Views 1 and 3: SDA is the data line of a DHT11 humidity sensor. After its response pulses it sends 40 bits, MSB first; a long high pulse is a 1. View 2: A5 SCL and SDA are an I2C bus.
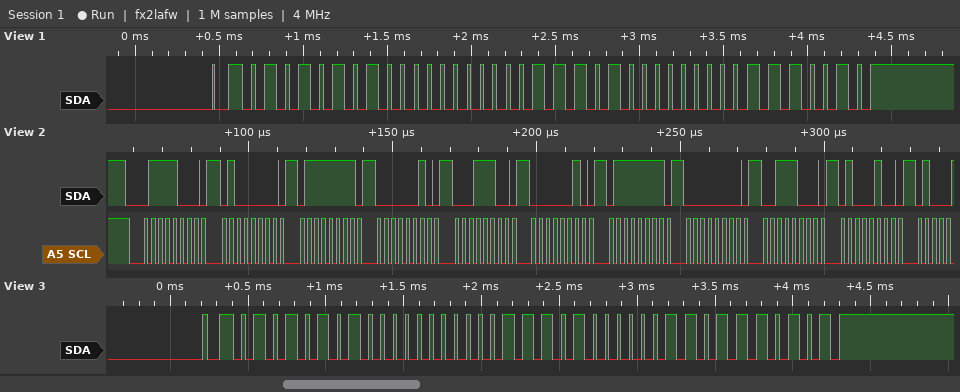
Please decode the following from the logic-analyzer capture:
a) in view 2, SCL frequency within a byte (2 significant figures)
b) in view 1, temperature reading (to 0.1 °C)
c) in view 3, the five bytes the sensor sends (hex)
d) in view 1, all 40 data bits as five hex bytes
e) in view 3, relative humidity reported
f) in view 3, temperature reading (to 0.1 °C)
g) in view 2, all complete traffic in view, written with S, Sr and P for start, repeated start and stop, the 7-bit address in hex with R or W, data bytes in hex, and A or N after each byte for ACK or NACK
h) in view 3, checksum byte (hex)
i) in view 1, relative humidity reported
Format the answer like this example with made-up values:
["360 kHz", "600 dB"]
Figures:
["400 kHz", "29.0 °C", "55 00 1D 03 75", "55 00 1D 00 72", "85 %", "29.3 °C", "S 3CW A 40 A 7F A 02 A 1C A 02 A 7F A 00 A 38 A 44 A", "0x75", "85 %"]
